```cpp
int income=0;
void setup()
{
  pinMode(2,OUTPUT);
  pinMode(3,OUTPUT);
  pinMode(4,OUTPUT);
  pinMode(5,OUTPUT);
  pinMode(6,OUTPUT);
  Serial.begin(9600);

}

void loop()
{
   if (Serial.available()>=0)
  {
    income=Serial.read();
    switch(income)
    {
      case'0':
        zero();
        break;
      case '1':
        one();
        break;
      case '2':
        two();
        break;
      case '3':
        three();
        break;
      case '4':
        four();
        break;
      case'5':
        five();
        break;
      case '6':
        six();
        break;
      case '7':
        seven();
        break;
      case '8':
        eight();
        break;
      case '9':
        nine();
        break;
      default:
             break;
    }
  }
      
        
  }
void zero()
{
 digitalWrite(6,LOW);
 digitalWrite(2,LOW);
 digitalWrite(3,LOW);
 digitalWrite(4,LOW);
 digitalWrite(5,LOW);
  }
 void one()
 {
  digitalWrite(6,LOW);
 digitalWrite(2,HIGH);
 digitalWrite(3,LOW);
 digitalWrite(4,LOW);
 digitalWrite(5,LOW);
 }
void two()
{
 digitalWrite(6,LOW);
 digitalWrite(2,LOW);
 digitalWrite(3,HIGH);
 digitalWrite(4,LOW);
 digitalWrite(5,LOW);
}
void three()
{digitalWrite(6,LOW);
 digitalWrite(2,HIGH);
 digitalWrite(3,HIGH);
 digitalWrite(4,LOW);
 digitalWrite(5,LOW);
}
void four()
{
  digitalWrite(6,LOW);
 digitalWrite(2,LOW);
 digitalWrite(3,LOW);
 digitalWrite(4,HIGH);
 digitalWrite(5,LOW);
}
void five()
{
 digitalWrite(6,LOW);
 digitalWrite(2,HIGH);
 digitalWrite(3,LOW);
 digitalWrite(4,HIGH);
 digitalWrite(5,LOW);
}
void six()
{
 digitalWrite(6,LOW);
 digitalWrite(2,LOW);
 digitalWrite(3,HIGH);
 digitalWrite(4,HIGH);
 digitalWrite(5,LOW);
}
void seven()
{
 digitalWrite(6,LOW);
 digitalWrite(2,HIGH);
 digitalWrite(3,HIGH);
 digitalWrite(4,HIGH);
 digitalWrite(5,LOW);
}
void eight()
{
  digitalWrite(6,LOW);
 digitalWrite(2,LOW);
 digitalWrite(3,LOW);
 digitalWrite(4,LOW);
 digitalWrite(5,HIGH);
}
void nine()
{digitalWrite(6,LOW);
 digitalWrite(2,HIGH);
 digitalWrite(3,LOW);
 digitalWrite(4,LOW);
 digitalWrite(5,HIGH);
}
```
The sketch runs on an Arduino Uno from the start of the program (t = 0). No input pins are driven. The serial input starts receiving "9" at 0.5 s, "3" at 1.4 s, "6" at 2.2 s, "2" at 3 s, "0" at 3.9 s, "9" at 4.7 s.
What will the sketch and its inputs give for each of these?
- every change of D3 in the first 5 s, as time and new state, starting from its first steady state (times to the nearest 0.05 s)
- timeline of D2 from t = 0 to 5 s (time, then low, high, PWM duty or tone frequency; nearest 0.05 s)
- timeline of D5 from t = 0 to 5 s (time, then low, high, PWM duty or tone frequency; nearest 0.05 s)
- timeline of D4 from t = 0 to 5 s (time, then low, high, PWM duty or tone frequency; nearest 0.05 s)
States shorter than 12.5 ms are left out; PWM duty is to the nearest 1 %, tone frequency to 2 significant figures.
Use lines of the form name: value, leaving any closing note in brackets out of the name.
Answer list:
every change of D3 in the first 5 s, as time and new state, starting from its first steady state: 0 s low; 1.4 s high; 3.9 s low
timeline of D2 from t = 0 to 5 s: 0 s low; 0.5 s high; 2.2 s low; 4.7 s high
timeline of D5 from t = 0 to 5 s: 0 s low; 0.5 s high; 1.4 s low; 4.7 s high
timeline of D4 from t = 0 to 5 s: 0 s low; 2.2 s high; 3 s low
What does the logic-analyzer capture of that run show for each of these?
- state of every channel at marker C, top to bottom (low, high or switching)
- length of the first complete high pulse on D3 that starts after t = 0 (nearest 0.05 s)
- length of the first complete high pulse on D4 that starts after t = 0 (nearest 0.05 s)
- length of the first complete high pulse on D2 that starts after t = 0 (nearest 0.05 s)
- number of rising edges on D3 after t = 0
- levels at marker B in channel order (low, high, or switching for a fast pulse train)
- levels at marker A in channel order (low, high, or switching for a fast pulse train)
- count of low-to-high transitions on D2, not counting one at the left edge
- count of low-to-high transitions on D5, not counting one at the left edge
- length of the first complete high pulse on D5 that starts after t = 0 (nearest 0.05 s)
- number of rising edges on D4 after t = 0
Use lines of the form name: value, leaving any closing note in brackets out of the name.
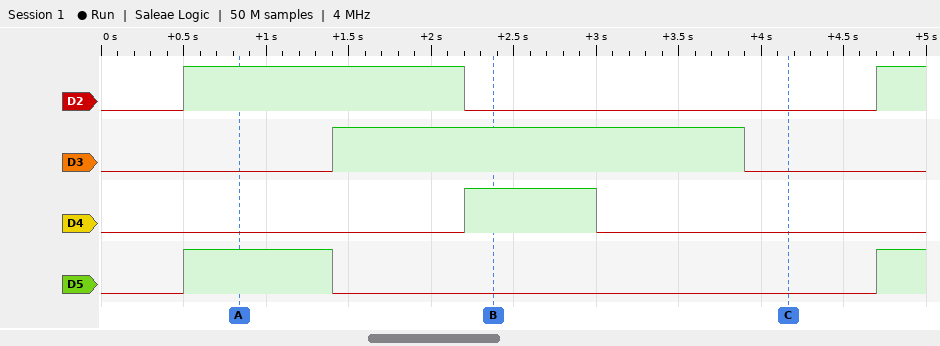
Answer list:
state of every channel at marker C, top to bottom: D2 low, D3 low, D4 low, D5 low
length of the first complete high pulse on D3 that starts after t = 0: 2.50 s
length of the first complete high pulse on D4 that starts after t = 0: 0.80 s
length of the first complete high pulse on D2 that starts after t = 0: 1.70 s
number of rising edges on D3 after t = 0: 1
levels at marker B in channel order: D2 low, D3 high, D4 high, D5 low
levels at marker A in channel order: D2 high, D3 low, D4 low, D5 high
count of low-to-high transitions on D2, not counting one at the left edge: 2
count of low-to-high transitions on D5, not counting one at the left edge: 2
length of the first complete high pulse on D5 that starts after t = 0: 0.90 s
number of rising edges on D4 after t = 0: 1
